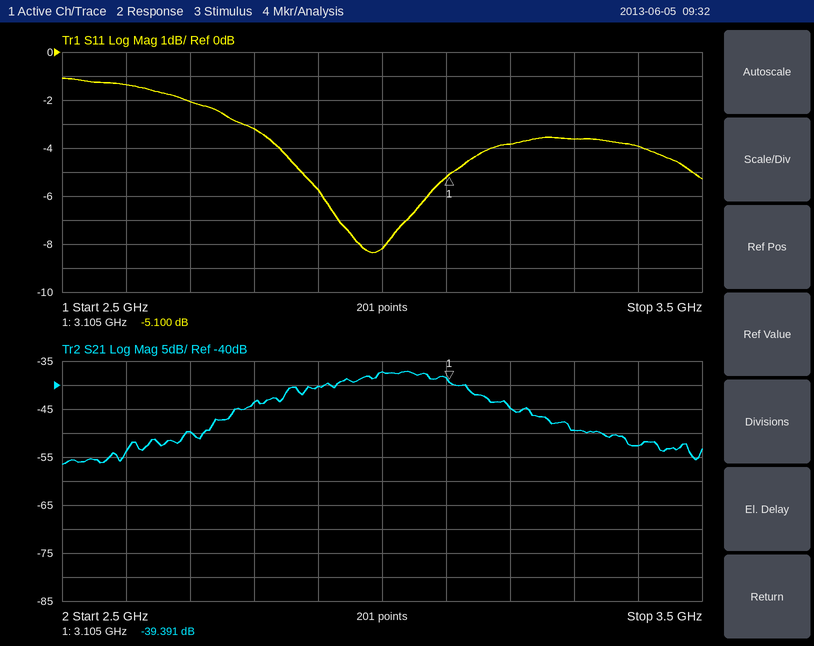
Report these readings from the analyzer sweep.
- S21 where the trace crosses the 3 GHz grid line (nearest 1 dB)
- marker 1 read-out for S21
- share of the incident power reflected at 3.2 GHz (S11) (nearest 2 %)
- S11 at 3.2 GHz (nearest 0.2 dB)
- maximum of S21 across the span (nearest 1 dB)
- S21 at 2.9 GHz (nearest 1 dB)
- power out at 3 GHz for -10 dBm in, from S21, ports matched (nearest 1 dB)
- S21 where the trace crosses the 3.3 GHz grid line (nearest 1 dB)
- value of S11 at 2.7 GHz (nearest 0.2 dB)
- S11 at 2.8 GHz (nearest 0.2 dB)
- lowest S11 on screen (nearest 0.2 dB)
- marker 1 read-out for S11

-37 dB
-39.391 dB
42 %
-3.8 dB
-37 dB
-40 dB
-47 dBm
-49 dB
-2.0 dB
-3.2 dB
-8.4 dB
-5.100 dB
